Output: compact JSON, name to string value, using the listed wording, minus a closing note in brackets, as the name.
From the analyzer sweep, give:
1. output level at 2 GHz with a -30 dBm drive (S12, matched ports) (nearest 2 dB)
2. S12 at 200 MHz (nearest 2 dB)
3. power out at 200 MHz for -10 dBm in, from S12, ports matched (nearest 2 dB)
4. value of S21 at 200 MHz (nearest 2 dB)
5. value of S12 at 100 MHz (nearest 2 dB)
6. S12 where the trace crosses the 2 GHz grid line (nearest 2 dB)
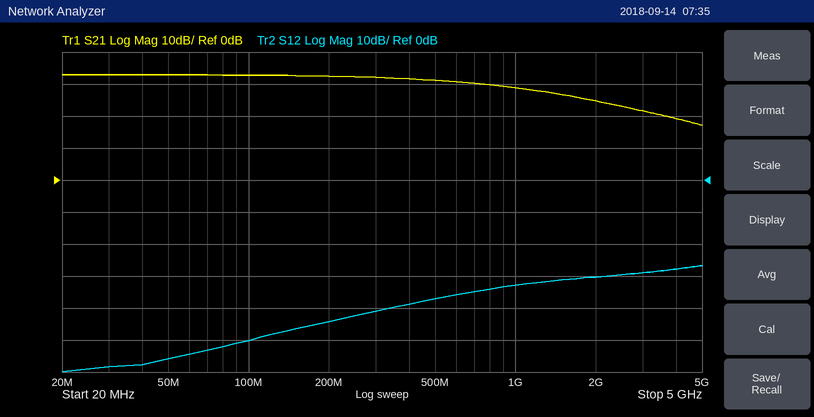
{"output level at 2 GHz with a -30 dBm drive (S12, matched ports)": "-60 dBm", "S12 at 200 MHz": "-44 dB", "power out at 200 MHz for -10 dBm in, from S12, ports matched": "-54 dBm", "value of S21 at 200 MHz": "32 dB", "value of S12 at 100 MHz": "-50 dB", "S12 where the trace crosses the 2 GHz grid line": "-30 dB"}
